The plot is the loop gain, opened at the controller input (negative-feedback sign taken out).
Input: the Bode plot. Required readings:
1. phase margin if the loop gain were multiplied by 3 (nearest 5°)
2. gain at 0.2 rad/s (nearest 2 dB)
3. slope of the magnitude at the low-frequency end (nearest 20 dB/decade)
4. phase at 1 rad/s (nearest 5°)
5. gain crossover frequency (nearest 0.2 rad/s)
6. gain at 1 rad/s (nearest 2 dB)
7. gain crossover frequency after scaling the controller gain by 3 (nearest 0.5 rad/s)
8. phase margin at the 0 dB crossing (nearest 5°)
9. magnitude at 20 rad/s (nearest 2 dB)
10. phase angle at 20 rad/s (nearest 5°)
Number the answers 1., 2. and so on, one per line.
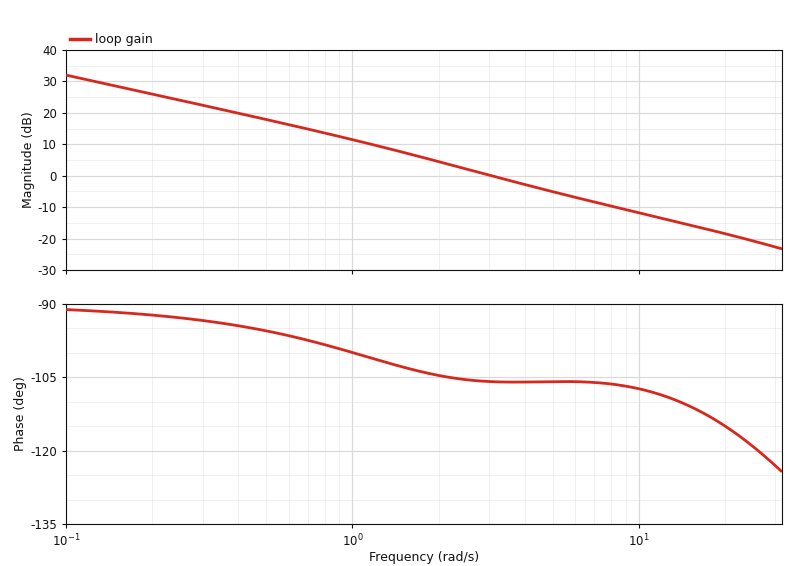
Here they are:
1. 75°
2. 26 dB
3. -20 dB/decade
4. -100°
5. 3.0 rad/s
6. 12 dB
7. 8.0 rad/s
8. 75°
9. -18 dB
10. -115°
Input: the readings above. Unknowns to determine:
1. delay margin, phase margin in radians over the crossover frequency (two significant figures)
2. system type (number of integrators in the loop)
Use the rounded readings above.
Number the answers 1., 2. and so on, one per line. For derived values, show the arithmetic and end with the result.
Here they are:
1. 75 × π / 180 / 3 = 0.44 s
2. 1
